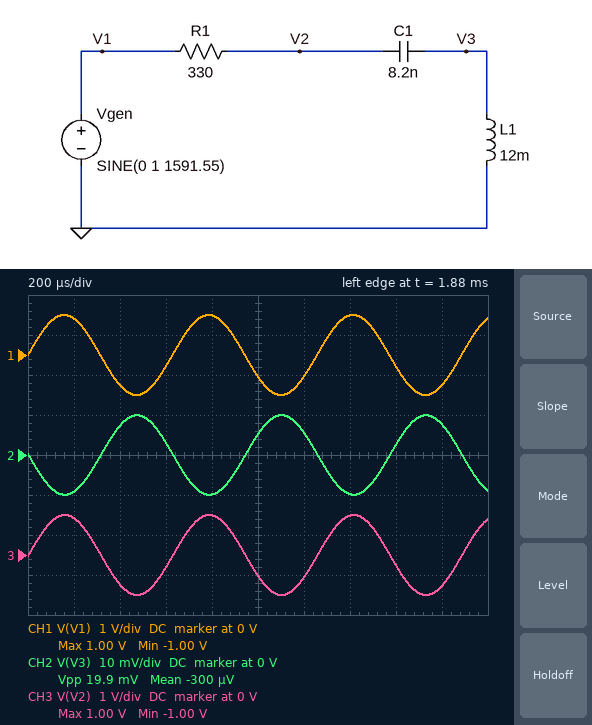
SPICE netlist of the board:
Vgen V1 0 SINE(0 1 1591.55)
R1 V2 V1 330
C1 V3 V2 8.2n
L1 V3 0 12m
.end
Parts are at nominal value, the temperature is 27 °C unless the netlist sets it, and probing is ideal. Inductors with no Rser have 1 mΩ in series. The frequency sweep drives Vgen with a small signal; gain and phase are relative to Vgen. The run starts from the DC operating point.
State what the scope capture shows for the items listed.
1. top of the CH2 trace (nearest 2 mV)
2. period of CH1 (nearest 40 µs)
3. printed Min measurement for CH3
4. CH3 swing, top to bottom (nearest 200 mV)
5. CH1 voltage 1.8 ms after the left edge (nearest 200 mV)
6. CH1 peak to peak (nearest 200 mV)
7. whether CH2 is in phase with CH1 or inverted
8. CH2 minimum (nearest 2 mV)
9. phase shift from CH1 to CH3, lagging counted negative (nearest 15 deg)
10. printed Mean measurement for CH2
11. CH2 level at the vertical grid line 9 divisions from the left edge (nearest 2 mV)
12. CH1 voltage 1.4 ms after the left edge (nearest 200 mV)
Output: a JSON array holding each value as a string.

["10 mV", "640 µs", "-1.00 V", "2.0 V", "-800 mV", "2.0 V", "inverted", "-10 mV", "0 deg", "-300 µV", "8 mV", "1.0 V"]
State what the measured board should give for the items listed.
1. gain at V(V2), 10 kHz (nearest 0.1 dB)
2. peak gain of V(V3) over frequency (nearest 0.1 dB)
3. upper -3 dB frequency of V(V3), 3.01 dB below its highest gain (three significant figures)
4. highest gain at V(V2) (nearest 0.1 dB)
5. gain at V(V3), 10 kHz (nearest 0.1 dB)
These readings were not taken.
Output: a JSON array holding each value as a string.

["-0.3 dB", "11.4 dB", "19.3 kHz", "0 dB", "-4.3 dB"]
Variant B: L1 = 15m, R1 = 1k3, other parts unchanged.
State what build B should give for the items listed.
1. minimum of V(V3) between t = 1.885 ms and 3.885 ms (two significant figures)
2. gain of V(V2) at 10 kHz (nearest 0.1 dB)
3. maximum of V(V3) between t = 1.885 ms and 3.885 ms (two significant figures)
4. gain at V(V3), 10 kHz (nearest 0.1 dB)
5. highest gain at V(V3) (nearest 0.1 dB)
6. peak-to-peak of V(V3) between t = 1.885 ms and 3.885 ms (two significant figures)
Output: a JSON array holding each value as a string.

["-12 mV", "-4.3 dB", "12 mV", "-4.8 dB", "1.5 dB", "25 mV"]
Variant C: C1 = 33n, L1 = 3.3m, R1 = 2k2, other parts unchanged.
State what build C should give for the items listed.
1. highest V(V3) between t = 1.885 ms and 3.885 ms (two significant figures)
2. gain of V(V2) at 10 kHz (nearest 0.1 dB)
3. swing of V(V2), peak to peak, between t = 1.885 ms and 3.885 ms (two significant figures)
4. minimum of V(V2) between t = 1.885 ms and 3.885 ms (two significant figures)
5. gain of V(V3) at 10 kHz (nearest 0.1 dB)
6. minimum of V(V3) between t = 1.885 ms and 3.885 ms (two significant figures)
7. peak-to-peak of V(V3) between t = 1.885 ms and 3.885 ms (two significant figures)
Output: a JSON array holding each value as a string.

["8.9 mV", "-18.1 dB", "1.6 V", "-810 mV", "-20.6 dB", "-8.9 mV", "18 mV"]
